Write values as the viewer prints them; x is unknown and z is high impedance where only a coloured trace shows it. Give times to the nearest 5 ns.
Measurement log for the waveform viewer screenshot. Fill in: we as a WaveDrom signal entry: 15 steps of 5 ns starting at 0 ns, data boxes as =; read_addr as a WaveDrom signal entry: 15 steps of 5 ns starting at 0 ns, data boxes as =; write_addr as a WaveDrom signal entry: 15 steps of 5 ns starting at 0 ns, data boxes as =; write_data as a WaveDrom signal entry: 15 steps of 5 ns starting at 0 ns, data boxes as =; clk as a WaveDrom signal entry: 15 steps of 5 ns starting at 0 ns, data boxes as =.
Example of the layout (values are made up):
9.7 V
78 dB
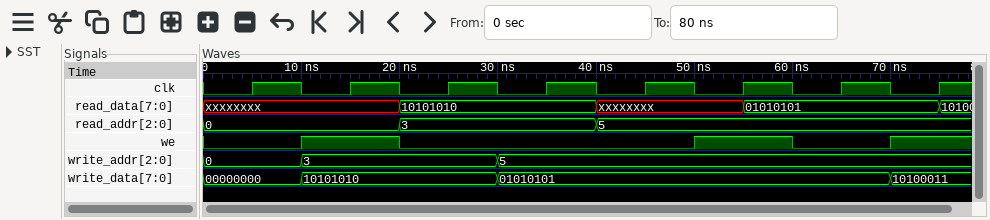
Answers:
{name: 'we', wave: '0.1.0.....1.0.1'}
{name: 'read_addr', wave: '=...=...=......', data: '0 3 5'}
{name: 'write_addr', wave: '=.=...=........', data: '0 3 5'}
{name: 'write_data', wave: '=.=...=.......=', data: '00000000 10101010 01010101 10100011'}
{name: 'clk', wave: '010101010101010'}
